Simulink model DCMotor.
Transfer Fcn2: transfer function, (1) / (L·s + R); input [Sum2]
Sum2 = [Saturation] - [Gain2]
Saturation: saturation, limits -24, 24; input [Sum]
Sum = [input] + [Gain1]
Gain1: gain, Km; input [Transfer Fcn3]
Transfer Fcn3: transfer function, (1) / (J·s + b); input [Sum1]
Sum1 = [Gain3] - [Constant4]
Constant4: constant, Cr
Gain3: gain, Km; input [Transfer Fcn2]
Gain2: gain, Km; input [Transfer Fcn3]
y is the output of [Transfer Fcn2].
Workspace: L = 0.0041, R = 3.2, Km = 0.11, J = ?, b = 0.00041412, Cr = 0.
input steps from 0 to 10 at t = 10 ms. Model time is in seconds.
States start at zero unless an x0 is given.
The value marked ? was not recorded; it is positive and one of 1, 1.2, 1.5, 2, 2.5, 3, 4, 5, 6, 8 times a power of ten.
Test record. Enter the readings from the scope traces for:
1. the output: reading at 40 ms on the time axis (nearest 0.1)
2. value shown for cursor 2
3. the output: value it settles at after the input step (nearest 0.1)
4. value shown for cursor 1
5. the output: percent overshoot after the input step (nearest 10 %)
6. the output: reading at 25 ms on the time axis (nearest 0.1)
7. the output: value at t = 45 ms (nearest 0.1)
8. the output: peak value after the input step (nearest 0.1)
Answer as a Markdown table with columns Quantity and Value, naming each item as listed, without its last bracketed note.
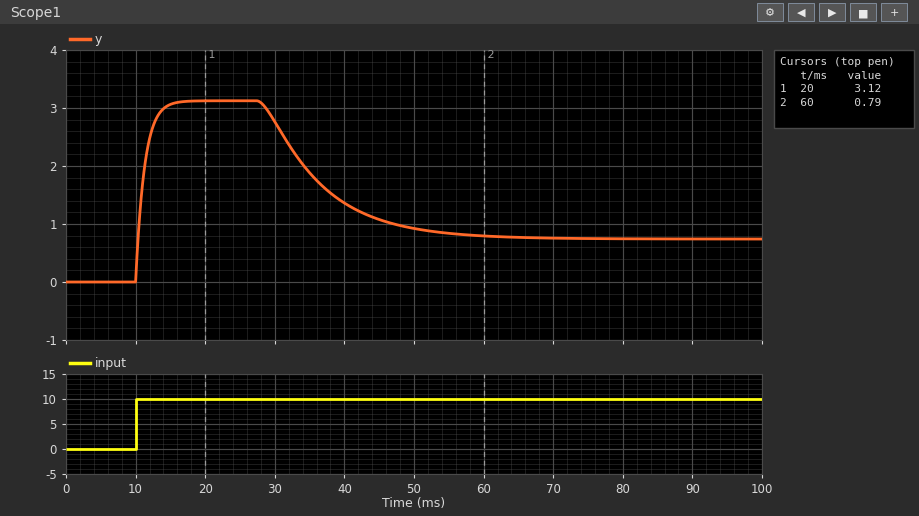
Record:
| Quantity | Value |
|---|---|
| the output: reading at 40 ms on the time axis | 1.4 |
| value shown for cursor 2 | 0.79 |
| the output: value it settles at after the input step | 0.7 |
| value shown for cursor 1 | 3.12 |
| the output: percent overshoot after the input step | 320 % |
| the output: reading at 25 ms on the time axis | 3.1 |
| the output: value at t = 45 ms | 1.1 |
| the output: peak value after the input step | 3.1 |
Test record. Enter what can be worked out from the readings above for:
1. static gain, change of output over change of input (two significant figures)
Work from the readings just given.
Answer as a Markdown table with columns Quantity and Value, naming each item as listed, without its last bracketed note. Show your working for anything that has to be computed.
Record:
| Quantity | Value |
|---|---|
| static gain, change of output over change of input | (0.7 - 0) / (10 - 0) = 0.070 |
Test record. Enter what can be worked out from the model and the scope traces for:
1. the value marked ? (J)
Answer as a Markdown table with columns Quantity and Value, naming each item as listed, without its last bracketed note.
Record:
| Quantity | Value |
|---|---|
| the value marked ? | 4e-05 |
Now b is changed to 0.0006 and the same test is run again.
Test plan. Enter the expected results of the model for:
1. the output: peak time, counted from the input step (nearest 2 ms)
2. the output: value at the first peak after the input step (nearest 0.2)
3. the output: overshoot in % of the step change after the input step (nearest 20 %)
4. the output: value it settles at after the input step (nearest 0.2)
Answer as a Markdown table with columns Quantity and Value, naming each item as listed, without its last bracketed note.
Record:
| Quantity | Value |
|---|---|
| the output: peak time, counted from the input step | 18 ms |
| the output: value at the first peak after the input step | 3.2 |
| the output: overshoot in % of the step change after the input step | 200 % |
| the output: value it settles at after the input step | 1.0 |
